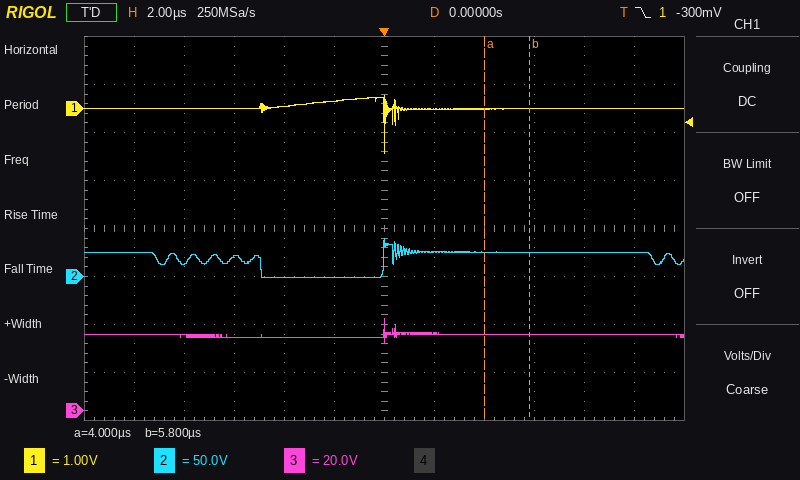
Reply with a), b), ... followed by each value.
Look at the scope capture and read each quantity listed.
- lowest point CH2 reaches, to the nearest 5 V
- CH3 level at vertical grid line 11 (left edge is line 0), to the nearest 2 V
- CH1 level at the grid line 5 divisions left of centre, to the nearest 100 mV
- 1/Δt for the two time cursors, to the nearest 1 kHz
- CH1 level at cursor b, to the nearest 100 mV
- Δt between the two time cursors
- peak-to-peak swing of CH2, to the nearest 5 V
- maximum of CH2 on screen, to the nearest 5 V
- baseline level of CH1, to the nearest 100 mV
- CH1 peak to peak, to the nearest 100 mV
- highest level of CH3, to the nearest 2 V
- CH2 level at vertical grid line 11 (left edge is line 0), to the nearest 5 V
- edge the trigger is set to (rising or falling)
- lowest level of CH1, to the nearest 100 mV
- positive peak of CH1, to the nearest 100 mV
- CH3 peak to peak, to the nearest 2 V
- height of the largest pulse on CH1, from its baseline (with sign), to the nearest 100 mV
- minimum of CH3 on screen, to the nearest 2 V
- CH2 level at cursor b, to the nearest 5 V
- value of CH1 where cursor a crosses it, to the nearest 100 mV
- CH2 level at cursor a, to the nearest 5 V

a) 0 V
b) 32 V
c) 0.0 V
d) 556 kHz
e) 0.0 V
f) 1.8 µs
g) 40 V
h) 40 V
i) 0.0 V
j) 1.2 V
k) 38 V
l) 25 V
m) falling
n) -900 mV
o) 300 mV
p) 10 V
q) -900 mV
r) 28 V
s) 25 V
t) 0.0 V
u) 25 V
